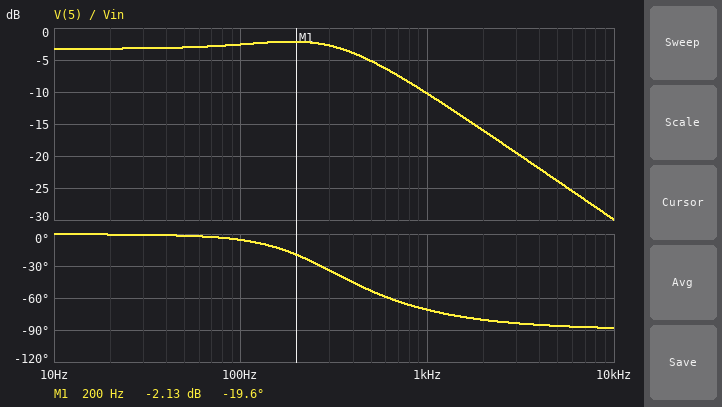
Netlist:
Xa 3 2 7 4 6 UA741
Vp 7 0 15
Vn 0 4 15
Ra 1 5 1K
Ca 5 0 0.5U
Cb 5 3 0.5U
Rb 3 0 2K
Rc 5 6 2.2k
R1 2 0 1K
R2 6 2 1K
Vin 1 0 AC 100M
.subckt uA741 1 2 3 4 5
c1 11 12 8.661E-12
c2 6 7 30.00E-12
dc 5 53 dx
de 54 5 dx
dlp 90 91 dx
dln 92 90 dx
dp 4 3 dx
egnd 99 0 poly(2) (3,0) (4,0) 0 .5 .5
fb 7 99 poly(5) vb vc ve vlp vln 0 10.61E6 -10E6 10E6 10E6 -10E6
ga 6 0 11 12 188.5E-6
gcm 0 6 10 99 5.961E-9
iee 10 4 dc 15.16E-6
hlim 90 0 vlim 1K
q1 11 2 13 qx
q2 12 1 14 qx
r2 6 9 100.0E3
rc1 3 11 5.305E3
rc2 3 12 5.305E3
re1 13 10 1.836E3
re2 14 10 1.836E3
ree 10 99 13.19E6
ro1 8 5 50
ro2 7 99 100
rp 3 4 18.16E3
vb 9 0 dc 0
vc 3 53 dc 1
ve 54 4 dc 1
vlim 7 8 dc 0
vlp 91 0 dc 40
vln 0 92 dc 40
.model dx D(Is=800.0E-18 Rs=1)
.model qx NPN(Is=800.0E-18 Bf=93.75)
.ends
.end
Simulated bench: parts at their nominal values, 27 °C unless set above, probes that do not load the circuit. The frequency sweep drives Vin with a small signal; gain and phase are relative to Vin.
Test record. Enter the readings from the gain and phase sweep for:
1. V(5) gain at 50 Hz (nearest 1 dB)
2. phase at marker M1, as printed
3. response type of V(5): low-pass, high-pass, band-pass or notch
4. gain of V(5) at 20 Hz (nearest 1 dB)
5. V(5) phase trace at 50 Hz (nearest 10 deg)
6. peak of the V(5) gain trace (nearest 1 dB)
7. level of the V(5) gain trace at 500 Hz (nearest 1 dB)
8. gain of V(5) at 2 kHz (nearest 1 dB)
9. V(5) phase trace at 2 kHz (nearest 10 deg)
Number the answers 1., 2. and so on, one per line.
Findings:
1. -3 dB
2. -19.6 deg
3. low-pass
4. -3 dB
5. 0 deg
6. -2 dB
7. -5 dB
8. -16 dB
9. -80 deg
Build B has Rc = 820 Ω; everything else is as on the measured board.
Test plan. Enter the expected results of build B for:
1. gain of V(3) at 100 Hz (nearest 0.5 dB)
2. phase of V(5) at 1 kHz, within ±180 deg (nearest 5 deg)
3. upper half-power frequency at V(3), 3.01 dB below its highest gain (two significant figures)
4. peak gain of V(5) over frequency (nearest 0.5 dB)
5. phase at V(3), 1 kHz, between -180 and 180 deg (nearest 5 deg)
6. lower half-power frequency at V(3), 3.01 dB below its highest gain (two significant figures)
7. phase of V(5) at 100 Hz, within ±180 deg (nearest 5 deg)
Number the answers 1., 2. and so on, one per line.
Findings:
1. -10.5 dB
2. -85 deg
3. 480 Hz
4. 3.0 dB
5. -75 deg
6. 230 Hz
7. 20 deg
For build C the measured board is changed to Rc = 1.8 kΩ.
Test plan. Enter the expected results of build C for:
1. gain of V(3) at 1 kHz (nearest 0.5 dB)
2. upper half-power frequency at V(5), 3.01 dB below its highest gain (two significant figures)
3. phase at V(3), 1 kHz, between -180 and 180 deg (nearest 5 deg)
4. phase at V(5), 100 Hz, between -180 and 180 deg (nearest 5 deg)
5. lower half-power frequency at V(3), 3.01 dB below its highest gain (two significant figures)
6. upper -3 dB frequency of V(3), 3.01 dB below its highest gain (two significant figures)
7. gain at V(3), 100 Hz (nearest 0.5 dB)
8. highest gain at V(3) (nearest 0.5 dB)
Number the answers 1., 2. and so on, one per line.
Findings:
1. -10.0 dB
2. 500 Hz
3. -65 deg
4. 0 deg
5. 130 Hz
6. 590 Hz
7. -8.5 dB
8. -3.0 dB
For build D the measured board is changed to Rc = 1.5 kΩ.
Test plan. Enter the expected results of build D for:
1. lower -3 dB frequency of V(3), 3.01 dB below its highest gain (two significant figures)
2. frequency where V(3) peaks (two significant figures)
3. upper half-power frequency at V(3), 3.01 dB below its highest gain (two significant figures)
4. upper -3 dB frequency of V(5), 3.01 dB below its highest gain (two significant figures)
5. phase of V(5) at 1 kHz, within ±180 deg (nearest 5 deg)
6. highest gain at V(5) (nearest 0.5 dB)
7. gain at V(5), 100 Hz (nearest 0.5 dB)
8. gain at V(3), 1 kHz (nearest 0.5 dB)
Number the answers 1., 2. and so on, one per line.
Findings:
1. 150 Hz
2. 290 Hz
3. 570 Hz
4. 500 Hz
5. -75 deg
6. -1.0 dB
7. -3.0 dB
8. -10.0 dB
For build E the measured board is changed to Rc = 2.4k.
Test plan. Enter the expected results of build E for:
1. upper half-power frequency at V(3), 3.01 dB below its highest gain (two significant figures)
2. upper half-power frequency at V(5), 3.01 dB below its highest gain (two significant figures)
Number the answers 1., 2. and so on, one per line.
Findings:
1. 620 Hz
2. 490 Hz
